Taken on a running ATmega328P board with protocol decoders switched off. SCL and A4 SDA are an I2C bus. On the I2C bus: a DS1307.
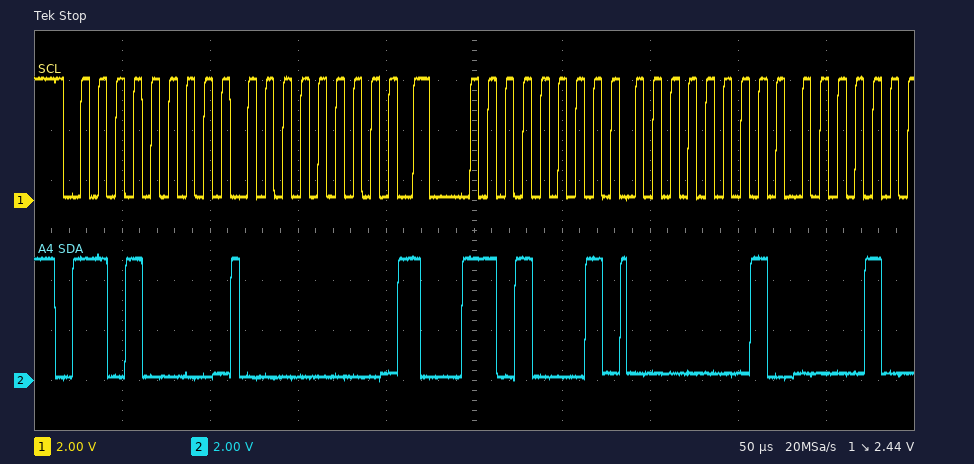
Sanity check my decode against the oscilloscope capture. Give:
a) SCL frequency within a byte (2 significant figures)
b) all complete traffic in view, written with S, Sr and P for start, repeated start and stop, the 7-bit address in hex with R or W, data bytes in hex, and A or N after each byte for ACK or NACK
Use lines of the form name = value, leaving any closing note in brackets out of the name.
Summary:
SCL frequency within a byte = 100 kHz
all complete traffic in view, written with S, Sr and P for start, repeated start and stop, the 7-bit address in hex with R or W, data bytes in hex, and A or N after each byte for ACK or NACK = S 68W A 00 A Sr 68R A 01 A
